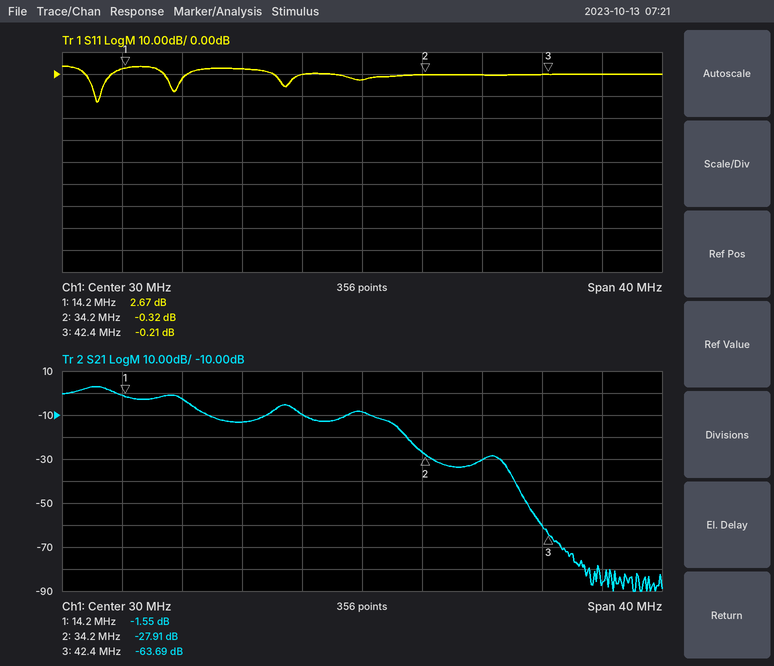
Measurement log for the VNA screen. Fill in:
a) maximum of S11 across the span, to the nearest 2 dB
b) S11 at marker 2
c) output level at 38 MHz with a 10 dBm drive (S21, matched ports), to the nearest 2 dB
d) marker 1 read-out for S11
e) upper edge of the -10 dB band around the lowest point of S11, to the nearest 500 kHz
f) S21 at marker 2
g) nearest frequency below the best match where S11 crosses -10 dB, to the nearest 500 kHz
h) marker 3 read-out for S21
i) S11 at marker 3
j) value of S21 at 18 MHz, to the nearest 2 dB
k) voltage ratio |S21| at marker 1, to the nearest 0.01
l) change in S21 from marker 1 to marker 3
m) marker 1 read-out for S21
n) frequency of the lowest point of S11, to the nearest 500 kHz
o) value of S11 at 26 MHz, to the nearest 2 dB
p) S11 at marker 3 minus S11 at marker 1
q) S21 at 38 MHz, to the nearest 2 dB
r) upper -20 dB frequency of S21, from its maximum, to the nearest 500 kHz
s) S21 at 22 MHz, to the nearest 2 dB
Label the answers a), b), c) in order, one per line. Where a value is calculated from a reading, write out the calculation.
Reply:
a) 4 dB
b) -0.32 dB
c) 10 dBm + (-30 dB) = -20 dBm
d) 2.67 dB
e) 12.5 MHz
f) -27.91 dB
g) 12.0 MHz
h) -63.69 dB
i) -0.21 dB
j) -2 dB
k) 10^(-1.55/20) ≈ 0.84
l) -63.69 − (-1.55) = -62.14 dB
m) -1.55 dB
n) 12.5 MHz
o) 0 dB
p) -0.21 − (2.67) = -2.88 dB
q) -30 dB
r) 32.5 MHz
s) -14 dB
